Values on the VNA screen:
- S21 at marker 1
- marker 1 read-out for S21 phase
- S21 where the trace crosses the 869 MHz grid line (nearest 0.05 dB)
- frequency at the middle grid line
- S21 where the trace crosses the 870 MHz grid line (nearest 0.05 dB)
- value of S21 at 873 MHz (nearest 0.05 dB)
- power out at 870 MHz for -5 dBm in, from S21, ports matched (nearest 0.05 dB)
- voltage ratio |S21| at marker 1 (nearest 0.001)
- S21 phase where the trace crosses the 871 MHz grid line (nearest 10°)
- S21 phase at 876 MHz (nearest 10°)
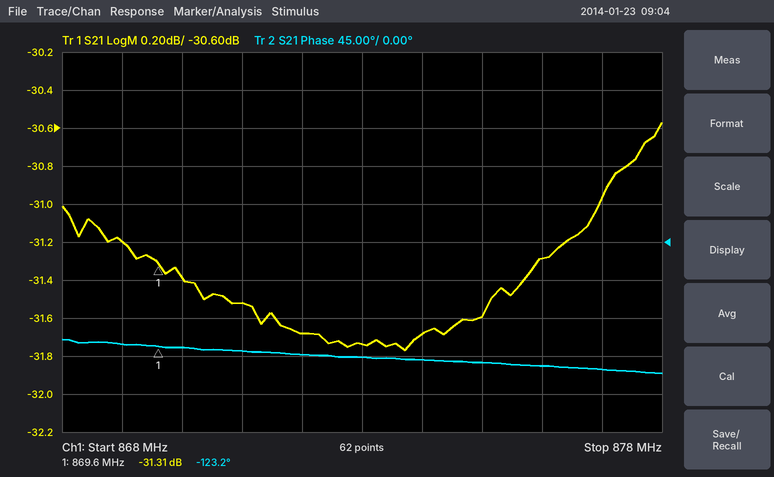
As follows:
-31.31 dB
-123.2°
-31.20 dB
873 MHz
-31.40 dB
-31.75 dB
-36.40 dBm
0.027
-130°
-150°
